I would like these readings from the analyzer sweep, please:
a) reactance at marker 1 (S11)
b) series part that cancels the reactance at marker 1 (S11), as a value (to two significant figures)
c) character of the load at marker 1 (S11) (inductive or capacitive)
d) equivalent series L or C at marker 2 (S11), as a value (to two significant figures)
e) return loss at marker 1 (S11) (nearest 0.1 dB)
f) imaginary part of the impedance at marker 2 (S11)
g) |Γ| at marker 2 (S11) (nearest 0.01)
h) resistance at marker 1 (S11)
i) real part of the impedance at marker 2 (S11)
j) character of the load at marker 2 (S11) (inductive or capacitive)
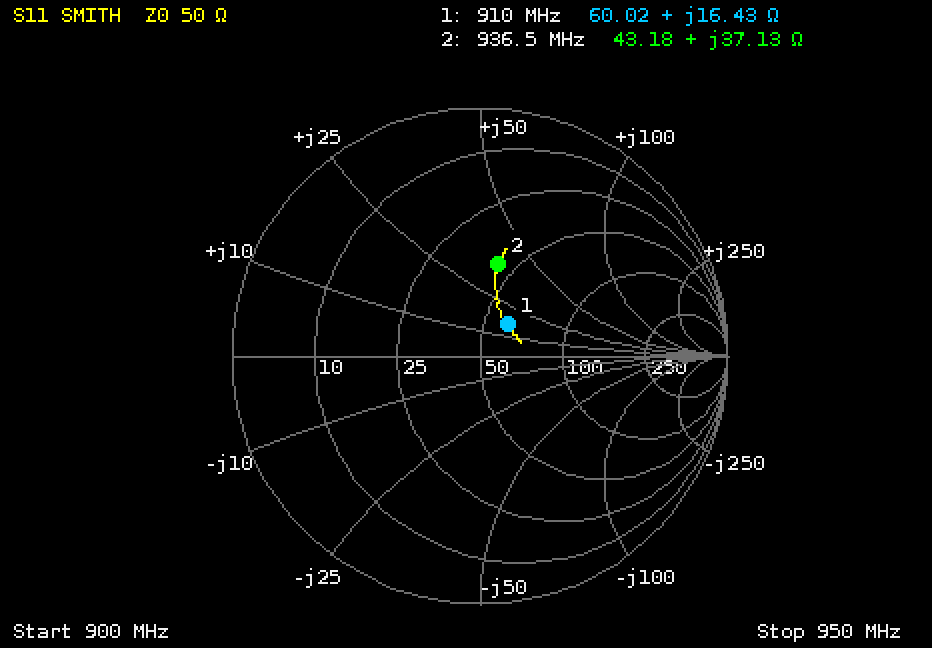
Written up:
+16.43 Ω
11 pF
inductive
6.3 nH
15.2 dB
+37.13 Ω
0.38
60.02 Ω
43.18 Ω
inductive
